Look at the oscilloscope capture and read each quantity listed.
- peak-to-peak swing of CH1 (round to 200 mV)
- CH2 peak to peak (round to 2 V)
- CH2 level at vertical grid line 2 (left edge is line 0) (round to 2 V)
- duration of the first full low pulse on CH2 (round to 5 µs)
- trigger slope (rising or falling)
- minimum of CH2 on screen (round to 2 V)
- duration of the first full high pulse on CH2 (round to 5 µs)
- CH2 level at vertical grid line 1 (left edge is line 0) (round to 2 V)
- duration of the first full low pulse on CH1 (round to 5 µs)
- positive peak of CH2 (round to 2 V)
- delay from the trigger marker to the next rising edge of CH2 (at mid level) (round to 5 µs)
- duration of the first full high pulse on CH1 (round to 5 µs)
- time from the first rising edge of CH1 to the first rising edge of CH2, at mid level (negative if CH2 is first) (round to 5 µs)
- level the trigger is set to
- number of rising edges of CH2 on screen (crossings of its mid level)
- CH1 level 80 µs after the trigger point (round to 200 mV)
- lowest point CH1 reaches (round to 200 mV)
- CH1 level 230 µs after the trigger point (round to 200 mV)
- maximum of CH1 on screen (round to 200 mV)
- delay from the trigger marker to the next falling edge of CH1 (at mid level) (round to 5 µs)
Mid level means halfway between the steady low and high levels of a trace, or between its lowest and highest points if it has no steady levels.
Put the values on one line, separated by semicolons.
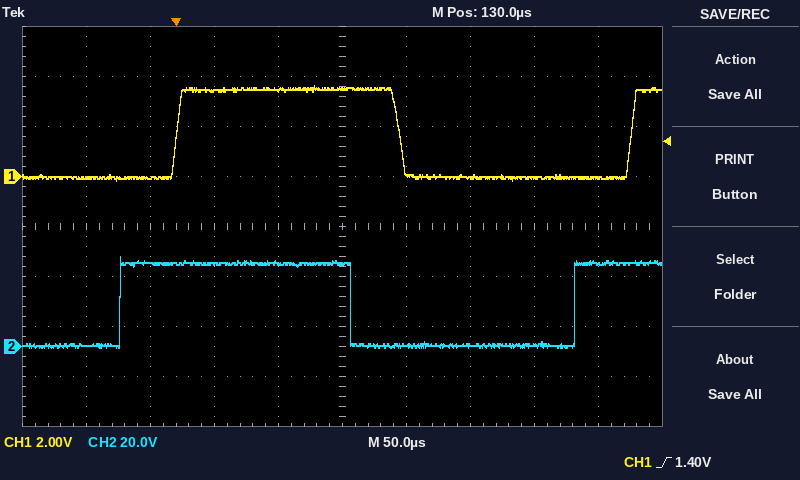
3.8 V; 36 V; 34 V; 175 µs; rising; 0 V; 180 µs; 0 V; 180 µs; 36 V; 310 µs; 175 µs; -45 µs; 1.40 V; 2; 3.4 V; -200 mV; 0.0 V; 3.6 V; 175 µs
